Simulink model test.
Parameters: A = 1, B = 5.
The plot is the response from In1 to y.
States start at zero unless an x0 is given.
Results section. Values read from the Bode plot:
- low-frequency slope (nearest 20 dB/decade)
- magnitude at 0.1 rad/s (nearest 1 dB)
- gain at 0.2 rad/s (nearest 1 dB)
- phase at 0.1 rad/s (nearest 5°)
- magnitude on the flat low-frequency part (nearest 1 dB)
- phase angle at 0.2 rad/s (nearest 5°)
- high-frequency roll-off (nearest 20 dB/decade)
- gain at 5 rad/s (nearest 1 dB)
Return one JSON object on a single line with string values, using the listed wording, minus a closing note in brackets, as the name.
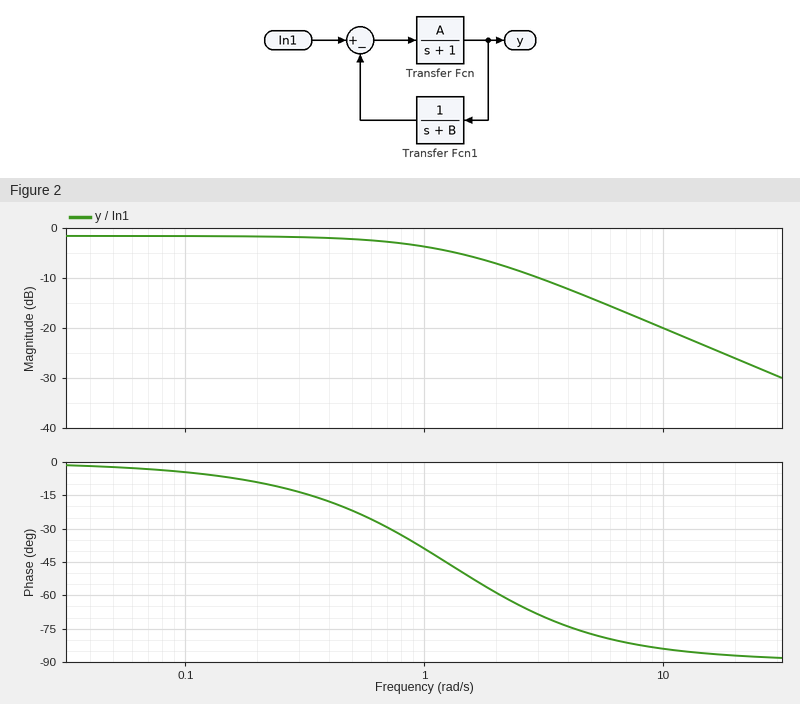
{"low-frequency slope": "0 dB/decade", "magnitude at 0.1 rad/s": "-2 dB", "gain at 0.2 rad/s": "-2 dB", "phase at 0.1 rad/s": "-5°", "magnitude on the flat low-frequency part": "-2 dB", "phase angle at 0.2 rad/s": "-10°", "high-frequency roll-off": "-20 dB/decade", "gain at 5 rad/s": "-14 dB"}
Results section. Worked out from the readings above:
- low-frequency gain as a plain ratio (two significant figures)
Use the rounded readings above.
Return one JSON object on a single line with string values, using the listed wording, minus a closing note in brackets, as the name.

{"low-frequency gain as a plain ratio": "0.79"}
